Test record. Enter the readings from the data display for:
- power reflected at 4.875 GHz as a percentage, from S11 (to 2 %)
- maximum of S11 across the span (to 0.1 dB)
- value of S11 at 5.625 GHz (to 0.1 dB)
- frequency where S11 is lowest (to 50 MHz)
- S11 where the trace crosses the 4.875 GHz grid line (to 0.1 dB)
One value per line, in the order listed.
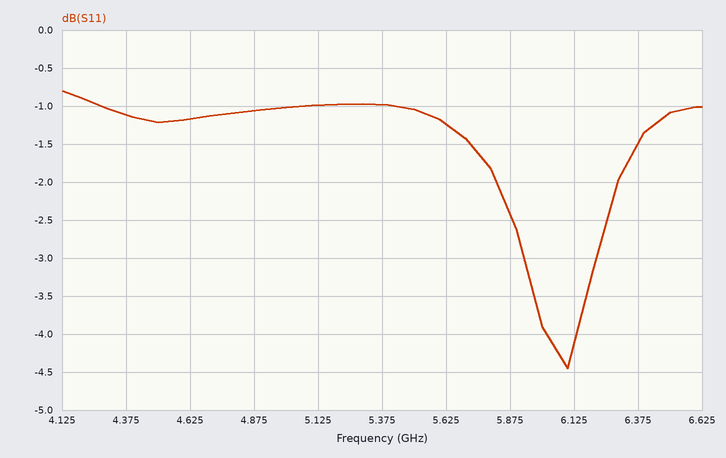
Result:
78 %
-0.8 dB
-1.2 dB
6.10 GHz
-1.1 dB
